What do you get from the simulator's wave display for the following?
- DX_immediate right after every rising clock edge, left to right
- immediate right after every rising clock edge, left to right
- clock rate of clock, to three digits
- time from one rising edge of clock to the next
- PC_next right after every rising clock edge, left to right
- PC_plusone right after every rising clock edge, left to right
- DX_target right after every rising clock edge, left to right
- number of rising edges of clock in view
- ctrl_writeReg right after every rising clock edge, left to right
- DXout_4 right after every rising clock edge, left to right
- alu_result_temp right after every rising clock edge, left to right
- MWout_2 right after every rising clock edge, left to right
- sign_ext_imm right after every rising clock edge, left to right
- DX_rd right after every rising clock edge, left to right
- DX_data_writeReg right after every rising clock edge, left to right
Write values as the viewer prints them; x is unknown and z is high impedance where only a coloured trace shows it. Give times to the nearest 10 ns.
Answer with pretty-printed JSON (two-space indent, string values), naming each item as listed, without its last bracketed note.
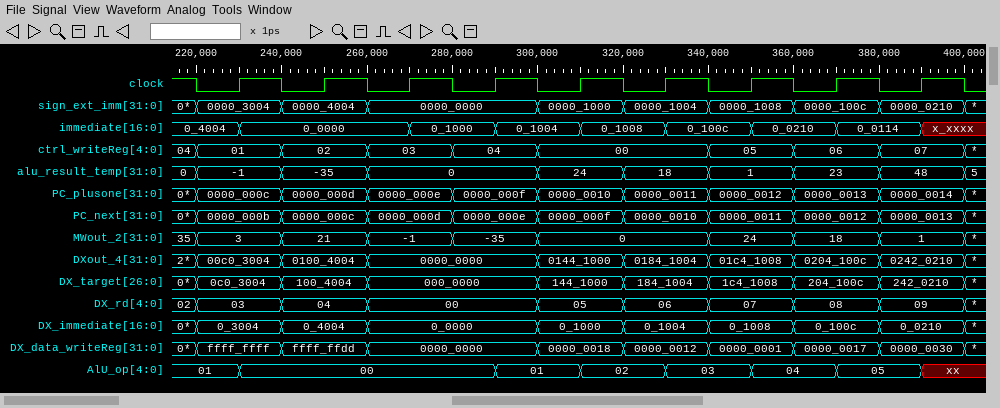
{
  "DX_immediate right after every rising clock edge, left to right": "0_3004, 0_4004, 0_0000, 0_0000, 0_1000, 0_1004, 0_1008, 0_100c, 0_0210",
  "immediate right after every rising clock edge, left to right": "0_0000, 0_0000, 0_1000, 0_1004, 0_1008, 0_100c, 0_0210, 0_0114, x_xxxx",
  "clock rate of clock, to three digits": "50.0 MHz",
  "time from one rising edge of clock to the next": "20 ns",
  "PC_next right after every rising clock edge, left to right": "0000_000b, 0000_000c, 0000_000d, 0000_000e, 0000_000f, 0000_0010, 0000_0011, 0000_0012, 0000_0013",
  "PC_plusone right after every rising clock edge, left to right": "0000_000c, 0000_000d, 0000_000e, 0000_000f, 0000_0010, 0000_0011, 0000_0012, 0000_0013, 0000_0014",
  "DX_target right after every rising clock edge, left to right": "0c0_3004, 100_4004, 000_0000, 000_0000, 144_1000, 184_1004, 1c4_1008, 204_100c, 242_0210",
  "number of rising edges of clock in view": "9",
  "ctrl_writeReg right after every rising clock edge, left to right": "01, 02, 03, 04, 00, 00, 05, 06, 07",
  "DXout_4 right after every rising clock edge, left to right": "00c0_3004, 0100_4004, 0000_0000, 0000_0000, 0144_1000, 0184_1004, 01c4_1008, 0204_100c, 0242_0210",
  "alu_result_temp right after every rising clock edge, left to right": "-1, -35, 0, 0, 24, 18, 1, 23, 48",
  "MWout_2 right after every rising clock edge, left to right": "3, 21, -1, -35, 0, 0, 24, 18, 1",
  "sign_ext_imm right after every rising clock edge, left to right": "0000_3004, 0000_4004, 0000_0000, 0000_0000, 0000_1000, 0000_1004, 0000_1008, 0000_100c, 0000_0210",
  "DX_rd right after every rising clock edge, left to right": "03, 04, 00, 00, 05, 06, 07, 08, 09",
  "DX_data_writeReg right after every rising clock edge, left to right": "ffff_ffff, ffff_ffdd, 0000_0000, 0000_0000, 0000_0018, 0000_0012, 0000_0001, 0000_0017, 0000_0030"
}
